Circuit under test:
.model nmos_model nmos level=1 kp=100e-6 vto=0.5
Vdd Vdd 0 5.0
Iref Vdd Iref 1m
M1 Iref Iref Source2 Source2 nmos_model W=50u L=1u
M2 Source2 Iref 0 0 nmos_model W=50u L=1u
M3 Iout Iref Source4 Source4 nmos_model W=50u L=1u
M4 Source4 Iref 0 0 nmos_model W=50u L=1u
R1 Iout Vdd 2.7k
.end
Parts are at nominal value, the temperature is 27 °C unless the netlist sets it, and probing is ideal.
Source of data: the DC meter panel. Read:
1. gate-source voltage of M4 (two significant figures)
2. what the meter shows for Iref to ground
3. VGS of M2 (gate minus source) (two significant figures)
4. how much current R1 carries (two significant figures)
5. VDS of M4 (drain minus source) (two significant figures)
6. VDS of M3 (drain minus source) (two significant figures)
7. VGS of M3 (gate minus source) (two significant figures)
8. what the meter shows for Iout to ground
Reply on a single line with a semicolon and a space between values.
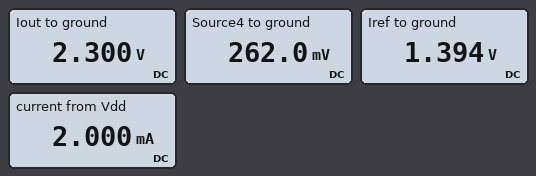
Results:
1.4 V; 1.394 V; 1.4 V; 1.0 mA; 260 mV; 2.0 V; 1.1 V; 2.300 V
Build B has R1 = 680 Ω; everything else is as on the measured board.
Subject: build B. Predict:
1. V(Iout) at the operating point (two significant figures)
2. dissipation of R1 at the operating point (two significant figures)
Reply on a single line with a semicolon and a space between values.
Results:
4.3 V; 680 µW
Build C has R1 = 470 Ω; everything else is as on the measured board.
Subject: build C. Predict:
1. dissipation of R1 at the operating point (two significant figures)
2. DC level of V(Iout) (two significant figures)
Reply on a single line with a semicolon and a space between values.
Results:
470 µW; 4.5 V
